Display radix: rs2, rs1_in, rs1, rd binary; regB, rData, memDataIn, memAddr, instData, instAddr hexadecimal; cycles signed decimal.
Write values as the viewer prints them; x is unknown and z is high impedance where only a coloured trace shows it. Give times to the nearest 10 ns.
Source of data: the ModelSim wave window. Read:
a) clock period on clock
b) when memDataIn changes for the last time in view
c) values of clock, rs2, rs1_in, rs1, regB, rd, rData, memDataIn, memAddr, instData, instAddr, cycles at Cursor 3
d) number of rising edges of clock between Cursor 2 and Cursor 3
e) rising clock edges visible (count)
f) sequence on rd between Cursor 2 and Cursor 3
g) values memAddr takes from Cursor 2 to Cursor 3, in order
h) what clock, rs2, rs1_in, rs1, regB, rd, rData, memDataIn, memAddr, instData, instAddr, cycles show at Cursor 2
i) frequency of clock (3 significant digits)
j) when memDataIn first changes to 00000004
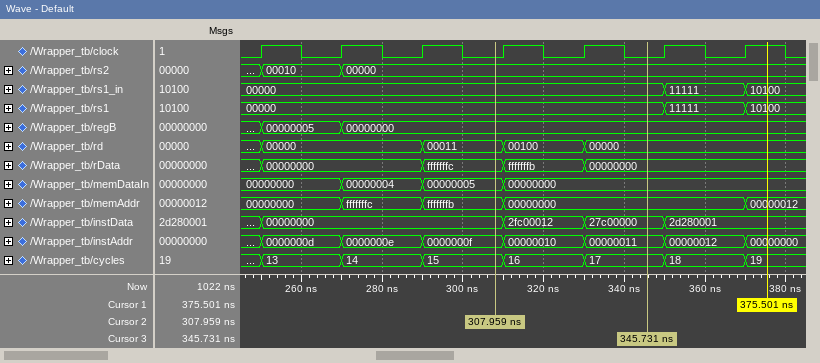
20 ns
310 ns
clock=0, rs2=00000, rs1_in=00000, rs1=00000, regB=00000000, rd=00000, rData=00000000, memDataIn=00000000, memAddr=00000000, instData=27c00000, instAddr=00000011, cycles=17
2
7
00011, 00100, 00000
fffffffb, 00000000
clock=0, rs2=00000, rs1_in=00000, rs1=00000, regB=00000000, rd=00011, rData=fffffffc, memDataIn=00000005, memAddr=fffffffb, instData=00000000, instAddr=0000000f, cycles=15
50.0 MHz
270 ns
